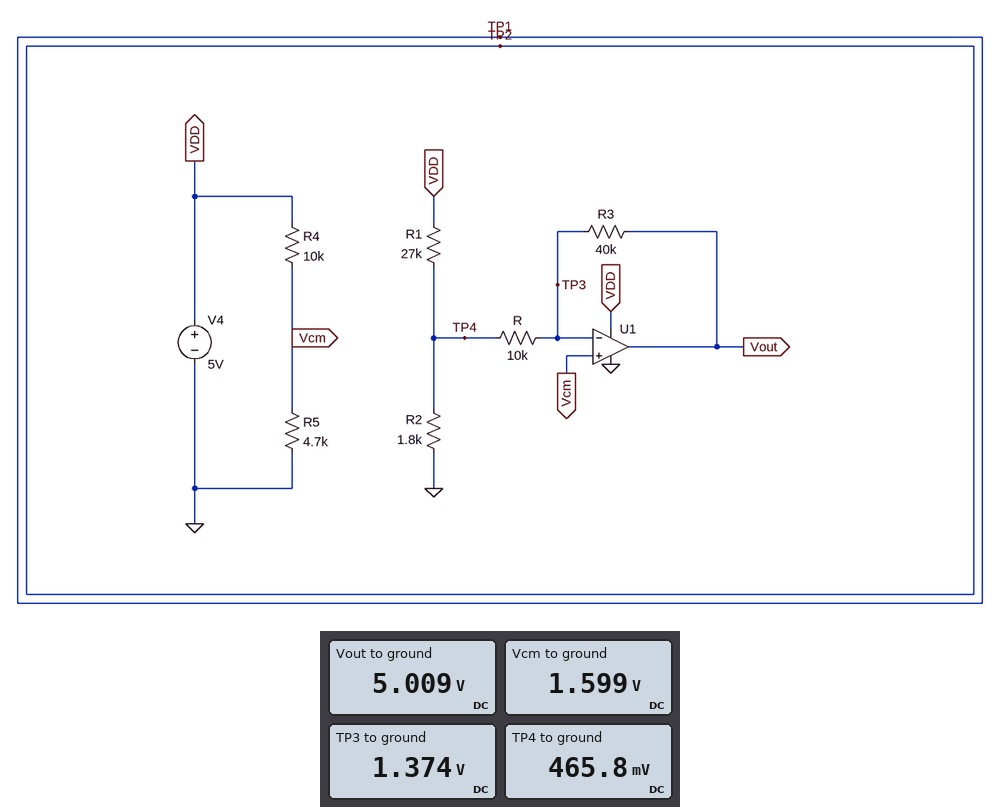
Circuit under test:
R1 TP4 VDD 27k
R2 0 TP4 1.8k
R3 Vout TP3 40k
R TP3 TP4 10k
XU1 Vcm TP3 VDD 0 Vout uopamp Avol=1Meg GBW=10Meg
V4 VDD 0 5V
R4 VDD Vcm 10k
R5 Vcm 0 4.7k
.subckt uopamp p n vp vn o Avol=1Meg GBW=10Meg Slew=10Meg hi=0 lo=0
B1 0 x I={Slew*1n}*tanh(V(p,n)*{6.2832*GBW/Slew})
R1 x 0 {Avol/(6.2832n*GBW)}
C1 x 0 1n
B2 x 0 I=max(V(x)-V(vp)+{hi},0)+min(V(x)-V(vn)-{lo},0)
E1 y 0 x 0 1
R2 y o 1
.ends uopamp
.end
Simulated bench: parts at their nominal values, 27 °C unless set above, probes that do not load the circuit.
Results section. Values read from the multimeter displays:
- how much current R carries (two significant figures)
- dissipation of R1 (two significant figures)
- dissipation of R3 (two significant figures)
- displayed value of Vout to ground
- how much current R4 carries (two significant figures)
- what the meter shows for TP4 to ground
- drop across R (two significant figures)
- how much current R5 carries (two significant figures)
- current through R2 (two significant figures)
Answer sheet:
91 µA
760 µW
330 µW
5.009 V
340 µA
465.8 mV
910 mV
340 µA
260 µA
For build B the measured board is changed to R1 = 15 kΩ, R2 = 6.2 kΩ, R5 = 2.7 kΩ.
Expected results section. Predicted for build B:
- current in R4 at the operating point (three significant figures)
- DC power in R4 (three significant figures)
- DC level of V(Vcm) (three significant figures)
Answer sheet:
394 µA
1.55 mW
1.06 V
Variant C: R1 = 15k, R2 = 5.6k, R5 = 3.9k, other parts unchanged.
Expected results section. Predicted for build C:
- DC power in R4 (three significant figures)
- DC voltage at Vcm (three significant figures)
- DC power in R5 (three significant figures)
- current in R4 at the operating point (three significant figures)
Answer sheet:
1.29 mW
1.40 V
505 µW
360 µA
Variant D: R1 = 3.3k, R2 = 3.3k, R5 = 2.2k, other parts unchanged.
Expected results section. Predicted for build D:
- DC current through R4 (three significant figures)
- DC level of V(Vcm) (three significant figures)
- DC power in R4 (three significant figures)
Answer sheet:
410 µA
902 mV
1.68 mW
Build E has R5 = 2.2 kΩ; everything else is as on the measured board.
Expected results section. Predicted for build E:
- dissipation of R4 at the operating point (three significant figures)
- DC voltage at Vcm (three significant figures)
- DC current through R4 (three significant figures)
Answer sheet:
1.68 mW
902 mV
410 µA
